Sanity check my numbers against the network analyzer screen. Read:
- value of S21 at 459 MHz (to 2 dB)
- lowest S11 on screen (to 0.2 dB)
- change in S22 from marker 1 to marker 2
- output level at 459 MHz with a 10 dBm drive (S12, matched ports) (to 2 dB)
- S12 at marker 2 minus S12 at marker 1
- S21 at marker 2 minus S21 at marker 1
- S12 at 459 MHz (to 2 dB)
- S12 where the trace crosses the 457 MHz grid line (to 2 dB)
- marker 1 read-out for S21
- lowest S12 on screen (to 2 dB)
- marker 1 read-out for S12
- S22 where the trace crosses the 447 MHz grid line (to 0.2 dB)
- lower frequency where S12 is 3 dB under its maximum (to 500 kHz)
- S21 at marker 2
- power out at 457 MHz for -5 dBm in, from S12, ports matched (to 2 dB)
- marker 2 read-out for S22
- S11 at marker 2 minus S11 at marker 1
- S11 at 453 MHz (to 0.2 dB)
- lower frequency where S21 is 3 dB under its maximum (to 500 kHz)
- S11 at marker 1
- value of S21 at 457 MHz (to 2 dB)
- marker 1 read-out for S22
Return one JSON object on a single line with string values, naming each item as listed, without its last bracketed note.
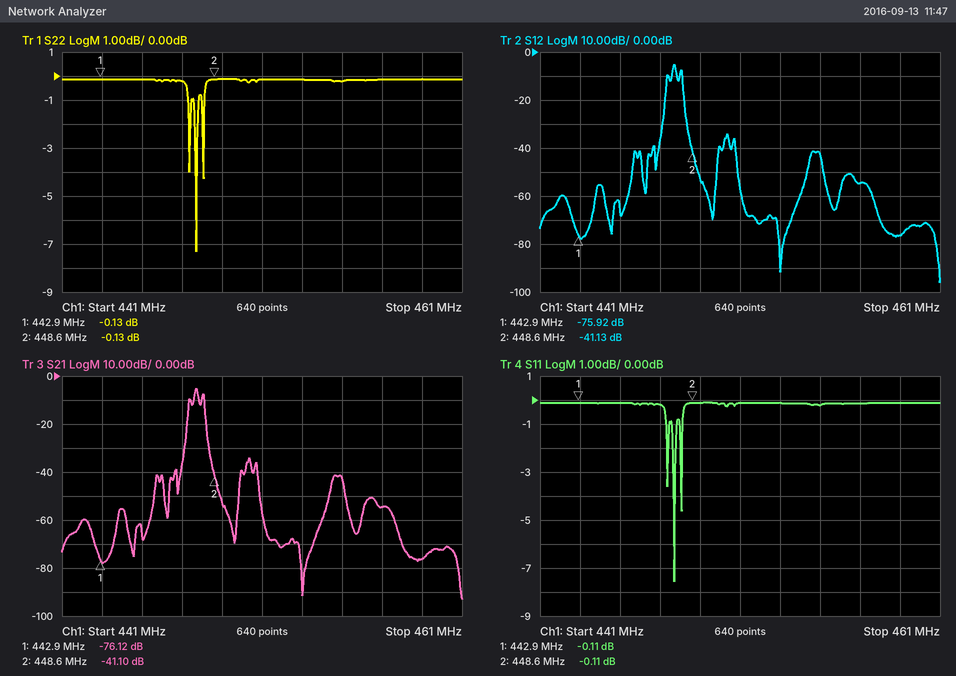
{"value of S21 at 459 MHz": "-76 dB", "lowest S11 on screen": "-7.6 dB", "change in S22 from marker 1 to marker 2": "0.00 dB", "output level at 459 MHz with a 10 dBm drive (S12, matched ports)": "-66 dBm", "S12 at marker 2 minus S12 at marker 1": "34.79 dB", "S21 at marker 2 minus S21 at marker 1": "35.02 dB", "S12 at 459 MHz": "-76 dB", "S12 where the trace crosses the 457 MHz grid line": "-54 dB", "marker 1 read-out for S21": "-76.12 dB", "lowest S12 on screen": "-96 dB", "marker 1 read-out for S12": "-75.92 dB", "S22 where the trace crosses the 447 MHz grid line": "-0.2 dB", "lower frequency where S12 is 3 dB under its maximum": "447.5 MHz", "S21 at marker 2": "-41.10 dB", "power out at 457 MHz for -5 dBm in, from S12, ports matched": "-60 dBm", "marker 2 read-out for S22": "-0.13 dB", "S11 at marker 2 minus S11 at marker 1": "0.00 dB", "S11 at 453 MHz": "-0.2 dB", "lower frequency where S21 is 3 dB under its maximum": "447.5 MHz", "S11 at marker 1": "-0.11 dB", "value of S21 at 457 MHz": "-54 dB", "marker 1 read-out for S22": "-0.13 dB"}
